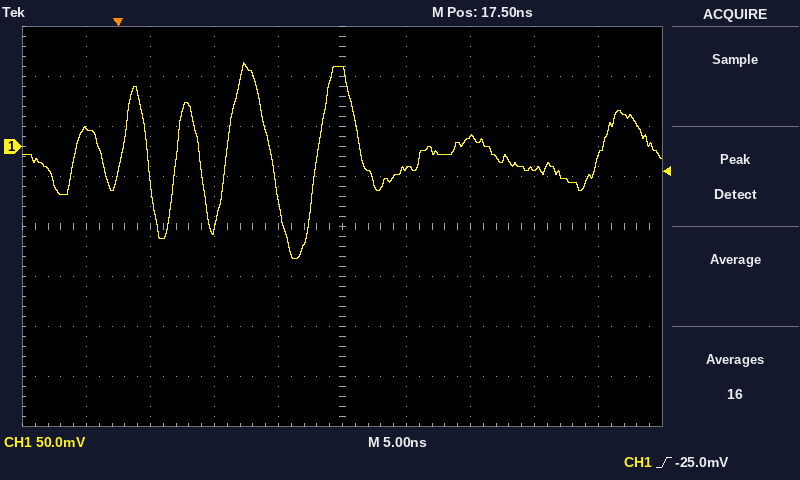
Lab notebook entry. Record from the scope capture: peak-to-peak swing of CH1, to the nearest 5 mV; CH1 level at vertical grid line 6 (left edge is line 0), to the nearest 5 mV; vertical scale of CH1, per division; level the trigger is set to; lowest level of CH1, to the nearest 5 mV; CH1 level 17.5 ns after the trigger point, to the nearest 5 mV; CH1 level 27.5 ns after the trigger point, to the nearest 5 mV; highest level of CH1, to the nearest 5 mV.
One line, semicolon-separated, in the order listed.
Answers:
195 mV; -20 mV; 50 mV; -25.0 mV; -110 mV; 75 mV; 10 mV; 85 mV
